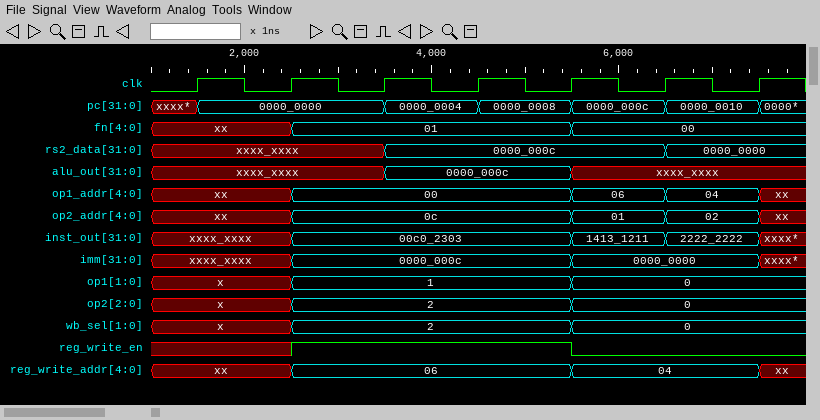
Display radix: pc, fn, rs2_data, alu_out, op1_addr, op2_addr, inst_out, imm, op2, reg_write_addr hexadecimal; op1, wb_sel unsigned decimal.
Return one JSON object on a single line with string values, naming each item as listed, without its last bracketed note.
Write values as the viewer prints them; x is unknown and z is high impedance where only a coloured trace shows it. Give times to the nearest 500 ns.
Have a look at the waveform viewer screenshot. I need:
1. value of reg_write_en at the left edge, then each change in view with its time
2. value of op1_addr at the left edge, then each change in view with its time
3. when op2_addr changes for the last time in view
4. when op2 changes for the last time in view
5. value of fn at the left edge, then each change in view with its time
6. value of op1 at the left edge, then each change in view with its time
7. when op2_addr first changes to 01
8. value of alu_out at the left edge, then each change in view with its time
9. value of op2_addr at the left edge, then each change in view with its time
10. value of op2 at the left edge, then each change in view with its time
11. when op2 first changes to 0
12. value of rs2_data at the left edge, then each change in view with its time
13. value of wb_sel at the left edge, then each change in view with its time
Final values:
{"value of reg_write_en at the left edge, then each change in view with its time": "x, 1 at 2500 ns, 0 at 5500 ns", "value of op1_addr at the left edge, then each change in view with its time": "xx, 00 at 2500 ns, 06 at 5500 ns, 04 at 6500 ns, xx at 7500 ns", "when op2_addr changes for the last time in view": "7500 ns", "when op2 changes for the last time in view": "5500 ns", "value of fn at the left edge, then each change in view with its time": "xx, 01 at 2500 ns, 00 at 5500 ns", "value of op1 at the left edge, then each change in view with its time": "x, 1 at 2500 ns, 0 at 5500 ns", "when op2_addr first changes to 01": "5500 ns", "value of alu_out at the left edge, then each change in view with its time": "xxxx_xxxx, 0000_000c at 3500 ns, xxxx_xxxx at 5500 ns", "value of op2_addr at the left edge, then each change in view with its time": "xx, 0c at 2500 ns, 01 at 5500 ns, 02 at 6500 ns, xx at 7500 ns", "value of op2 at the left edge, then each change in view with its time": "x, 2 at 2500 ns, 0 at 5500 ns", "when op2 first changes to 0": "5500 ns", "value of rs2_data at the left edge, then each change in view with its time": "xxxx_xxxx, 0000_000c at 3500 ns, 0000_0000 at 6500 ns", "value of wb_sel at the left edge, then each change in view with its time": "x, 2 at 2500 ns, 0 at 5500 ns"}
